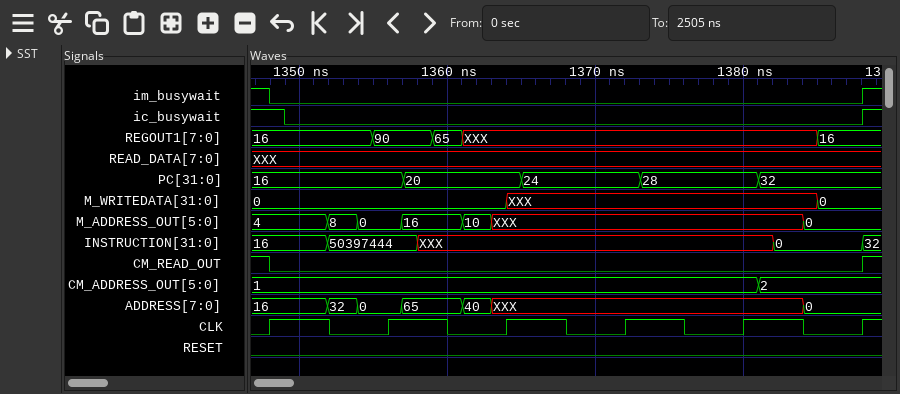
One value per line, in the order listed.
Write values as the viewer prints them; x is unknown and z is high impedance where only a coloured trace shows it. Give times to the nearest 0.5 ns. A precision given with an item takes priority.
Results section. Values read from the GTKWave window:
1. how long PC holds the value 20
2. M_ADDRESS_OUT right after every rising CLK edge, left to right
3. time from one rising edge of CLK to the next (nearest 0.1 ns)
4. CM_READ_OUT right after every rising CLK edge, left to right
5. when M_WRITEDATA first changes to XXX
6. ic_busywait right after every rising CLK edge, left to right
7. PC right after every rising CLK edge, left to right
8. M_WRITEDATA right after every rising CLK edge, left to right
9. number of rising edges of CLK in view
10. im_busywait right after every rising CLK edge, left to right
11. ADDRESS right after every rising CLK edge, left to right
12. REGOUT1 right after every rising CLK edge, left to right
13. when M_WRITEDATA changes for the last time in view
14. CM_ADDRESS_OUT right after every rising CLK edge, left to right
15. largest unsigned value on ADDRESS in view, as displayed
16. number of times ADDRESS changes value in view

8 ns
4, 0, XXX, XXX, XXX, 0
8 ns
0 0 0 0 0 1
1364 ns
1 0 0 0 0 1
16, 16, 20, 24, 28, 32
0, 0, XXX, XXX, XXX, 0
6
0 0 0 0 0 1
16, 0, XXX, XXX, XXX, 0
16, 90, XXX, XXX, XXX, 16
1385 ns
1, 1, 1, 1, 1, 2
65
6
